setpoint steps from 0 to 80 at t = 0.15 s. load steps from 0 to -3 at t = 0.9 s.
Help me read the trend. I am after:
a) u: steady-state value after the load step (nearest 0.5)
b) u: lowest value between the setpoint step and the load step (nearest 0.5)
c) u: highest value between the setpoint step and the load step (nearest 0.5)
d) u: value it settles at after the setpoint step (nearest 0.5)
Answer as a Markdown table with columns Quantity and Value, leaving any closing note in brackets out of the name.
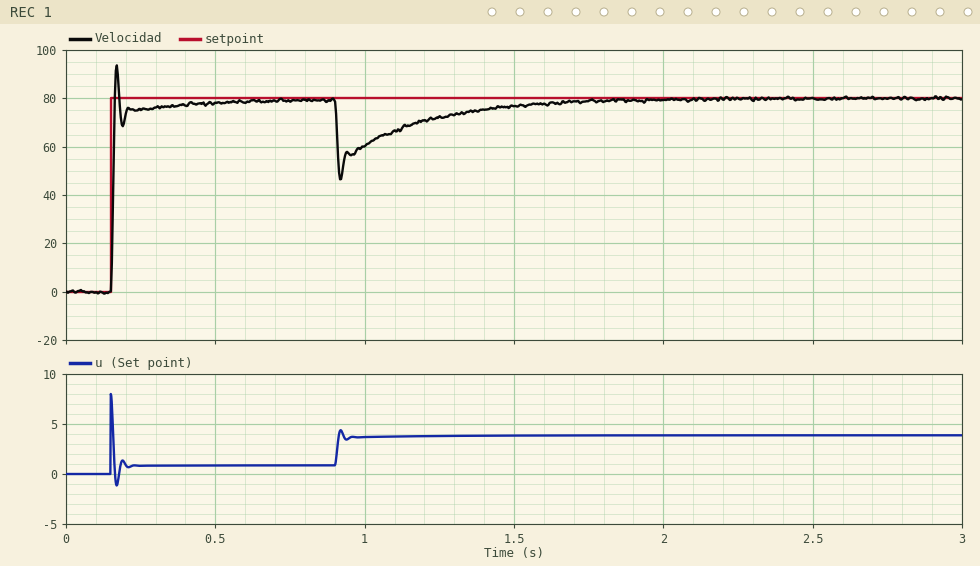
| Quantity | Value |
|---|---|
| u: steady-state value after the load step | 4.0 |
| u: lowest value between the setpoint step and the load step | -1.0 |
| u: highest value between the setpoint step and the load step | 8.0 |
| u: value it settles at after the setpoint step | 1.0 |
